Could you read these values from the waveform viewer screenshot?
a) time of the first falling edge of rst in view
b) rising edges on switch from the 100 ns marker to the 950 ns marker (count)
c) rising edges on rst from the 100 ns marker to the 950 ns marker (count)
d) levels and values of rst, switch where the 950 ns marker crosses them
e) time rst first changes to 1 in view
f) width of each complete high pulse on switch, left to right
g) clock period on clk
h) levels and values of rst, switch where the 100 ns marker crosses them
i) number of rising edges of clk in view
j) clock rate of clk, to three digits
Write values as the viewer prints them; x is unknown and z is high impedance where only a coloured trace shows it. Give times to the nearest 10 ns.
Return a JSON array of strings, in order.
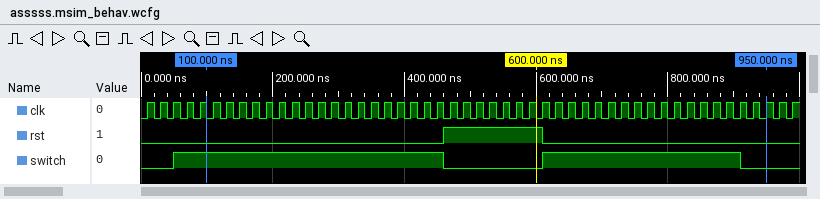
["610 ns", "1", "1", "rst=0, switch=0", "460 ns", "410 ns, 300 ns", "20 ns", "rst=0, switch=1", "50", "50.0 MHz"]
